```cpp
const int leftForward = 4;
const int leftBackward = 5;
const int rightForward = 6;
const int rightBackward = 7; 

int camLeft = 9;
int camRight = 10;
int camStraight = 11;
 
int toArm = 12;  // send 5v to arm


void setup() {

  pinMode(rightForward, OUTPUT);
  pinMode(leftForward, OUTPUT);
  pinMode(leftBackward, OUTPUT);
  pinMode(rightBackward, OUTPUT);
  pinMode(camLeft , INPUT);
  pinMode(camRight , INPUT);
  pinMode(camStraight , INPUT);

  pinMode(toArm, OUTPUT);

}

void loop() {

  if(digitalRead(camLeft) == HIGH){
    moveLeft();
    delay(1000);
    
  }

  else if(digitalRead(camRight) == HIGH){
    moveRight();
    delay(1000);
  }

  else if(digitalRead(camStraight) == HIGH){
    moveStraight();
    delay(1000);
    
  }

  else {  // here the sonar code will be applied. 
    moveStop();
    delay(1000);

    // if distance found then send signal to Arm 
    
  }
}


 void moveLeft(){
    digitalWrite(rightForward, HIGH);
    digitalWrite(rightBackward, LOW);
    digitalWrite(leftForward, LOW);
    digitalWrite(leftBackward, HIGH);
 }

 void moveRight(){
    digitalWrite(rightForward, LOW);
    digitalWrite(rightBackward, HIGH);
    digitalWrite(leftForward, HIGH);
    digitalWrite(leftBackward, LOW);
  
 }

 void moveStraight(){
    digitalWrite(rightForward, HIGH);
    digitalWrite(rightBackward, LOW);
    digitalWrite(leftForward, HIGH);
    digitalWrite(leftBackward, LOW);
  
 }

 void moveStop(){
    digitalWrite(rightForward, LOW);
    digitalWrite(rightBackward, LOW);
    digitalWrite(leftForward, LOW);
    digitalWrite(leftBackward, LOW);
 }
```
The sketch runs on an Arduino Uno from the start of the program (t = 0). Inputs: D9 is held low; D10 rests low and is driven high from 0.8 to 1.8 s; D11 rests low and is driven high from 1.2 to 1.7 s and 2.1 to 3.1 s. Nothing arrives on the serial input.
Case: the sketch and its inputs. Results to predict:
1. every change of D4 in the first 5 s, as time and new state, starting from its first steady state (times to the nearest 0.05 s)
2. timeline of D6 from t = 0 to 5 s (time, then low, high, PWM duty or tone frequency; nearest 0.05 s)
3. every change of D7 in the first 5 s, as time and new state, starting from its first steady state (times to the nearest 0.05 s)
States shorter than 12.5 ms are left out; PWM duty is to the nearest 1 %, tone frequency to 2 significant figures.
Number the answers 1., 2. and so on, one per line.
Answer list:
1. 0 s low; 1 s high; 2 s low; 3 s high; 4 s low
2. 0 s low; 3 s high; 4 s low
3. 0 s low; 1 s high; 2 s low
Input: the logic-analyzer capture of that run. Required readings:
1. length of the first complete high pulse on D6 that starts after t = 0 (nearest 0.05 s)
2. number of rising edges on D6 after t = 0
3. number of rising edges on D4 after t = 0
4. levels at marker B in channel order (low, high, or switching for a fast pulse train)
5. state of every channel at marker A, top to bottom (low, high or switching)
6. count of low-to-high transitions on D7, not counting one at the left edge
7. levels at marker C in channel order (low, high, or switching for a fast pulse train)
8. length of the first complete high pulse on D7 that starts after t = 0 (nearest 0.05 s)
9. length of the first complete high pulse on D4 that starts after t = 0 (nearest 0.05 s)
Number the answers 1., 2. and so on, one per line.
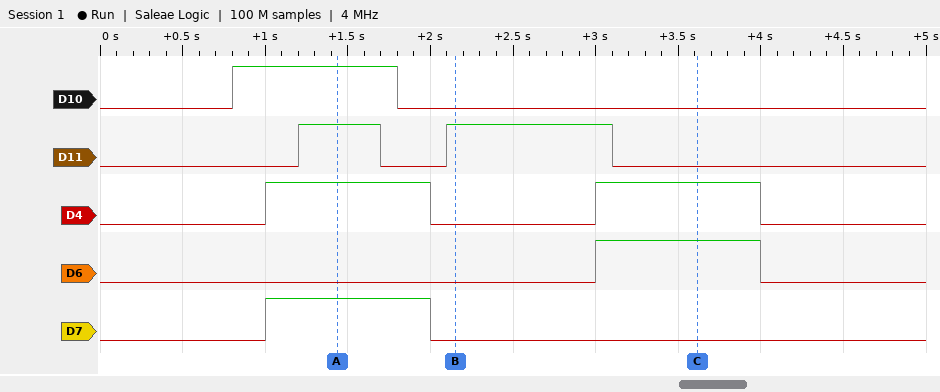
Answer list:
1. 1.00 s
2. 1
3. 2
4. D10 low, D11 high, D4 low, D6 low, D7 low
5. D10 high, D11 high, D4 high, D6 low, D7 high
6. 1
7. D10 low, D11 low, D4 high, D6 high, D7 low
8. 1.00 s
9. 1.00 s
